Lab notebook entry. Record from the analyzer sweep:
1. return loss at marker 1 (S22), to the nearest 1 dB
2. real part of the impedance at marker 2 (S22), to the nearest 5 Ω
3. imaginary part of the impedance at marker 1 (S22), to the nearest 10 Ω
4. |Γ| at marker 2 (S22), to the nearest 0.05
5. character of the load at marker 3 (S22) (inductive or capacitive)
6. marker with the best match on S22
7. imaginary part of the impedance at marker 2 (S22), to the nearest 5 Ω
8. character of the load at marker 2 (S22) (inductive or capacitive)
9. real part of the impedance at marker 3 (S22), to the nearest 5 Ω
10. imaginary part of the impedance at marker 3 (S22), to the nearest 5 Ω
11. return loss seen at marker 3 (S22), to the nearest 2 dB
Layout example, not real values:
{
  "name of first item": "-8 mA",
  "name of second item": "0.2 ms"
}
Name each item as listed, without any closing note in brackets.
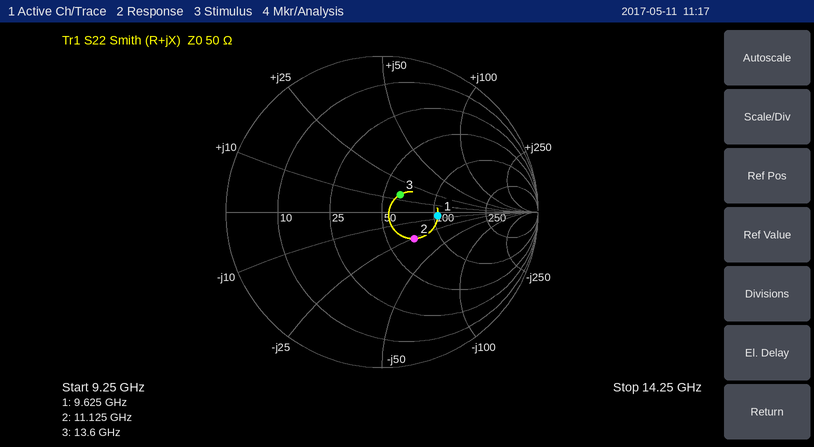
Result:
{
  "return loss at marker 1 (S22), to the nearest 1 dB": "9 dB",
  "real part of the impedance at marker 2 (S22), to the nearest 5 Ω": "70 Ω",
  "imaginary part of the impedance at marker 1 (S22), to the nearest 10 Ω": "-10 Ω",
  "|Γ| at marker 2 (S22), to the nearest 0.05": "0.25",
  "character of the load at marker 3 (S22)": "inductive",
  "marker with the best match on S22": "marker 3",
  "imaginary part of the impedance at marker 2 (S22), to the nearest 5 Ω": "-25 Ω",
  "character of the load at marker 2 (S22)": "capacitive",
  "real part of the impedance at marker 3 (S22), to the nearest 5 Ω": "60 Ω",
  "imaginary part of the impedance at marker 3 (S22), to the nearest 5 Ω": "+15 Ω",
  "return loss seen at marker 3 (S22), to the nearest 2 dB": "16 dB"
}
